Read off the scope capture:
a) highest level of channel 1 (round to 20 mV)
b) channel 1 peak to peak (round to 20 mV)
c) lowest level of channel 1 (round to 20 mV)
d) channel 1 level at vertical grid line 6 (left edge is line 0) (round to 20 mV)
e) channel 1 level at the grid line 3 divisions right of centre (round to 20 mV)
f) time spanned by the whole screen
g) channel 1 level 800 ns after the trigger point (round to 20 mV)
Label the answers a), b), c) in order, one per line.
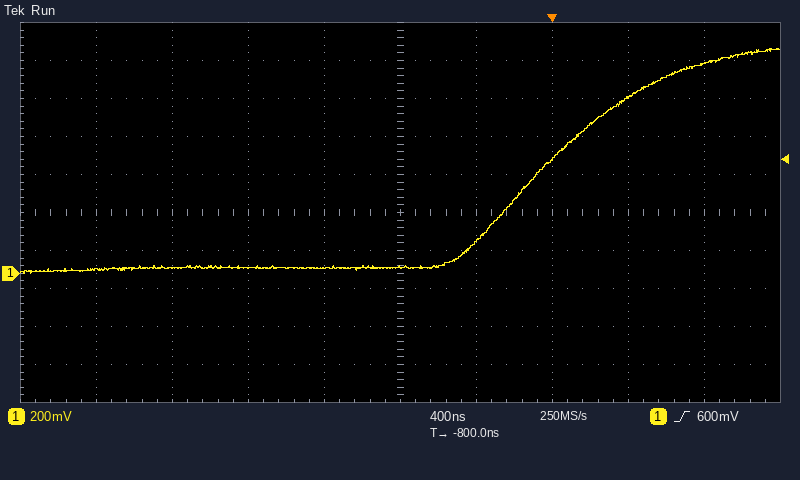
a) 1.18 V
b) 1.18 V
c) 0 mV
d) 160 mV
e) 920 mV
f) 4 µs
g) 1.10 V
